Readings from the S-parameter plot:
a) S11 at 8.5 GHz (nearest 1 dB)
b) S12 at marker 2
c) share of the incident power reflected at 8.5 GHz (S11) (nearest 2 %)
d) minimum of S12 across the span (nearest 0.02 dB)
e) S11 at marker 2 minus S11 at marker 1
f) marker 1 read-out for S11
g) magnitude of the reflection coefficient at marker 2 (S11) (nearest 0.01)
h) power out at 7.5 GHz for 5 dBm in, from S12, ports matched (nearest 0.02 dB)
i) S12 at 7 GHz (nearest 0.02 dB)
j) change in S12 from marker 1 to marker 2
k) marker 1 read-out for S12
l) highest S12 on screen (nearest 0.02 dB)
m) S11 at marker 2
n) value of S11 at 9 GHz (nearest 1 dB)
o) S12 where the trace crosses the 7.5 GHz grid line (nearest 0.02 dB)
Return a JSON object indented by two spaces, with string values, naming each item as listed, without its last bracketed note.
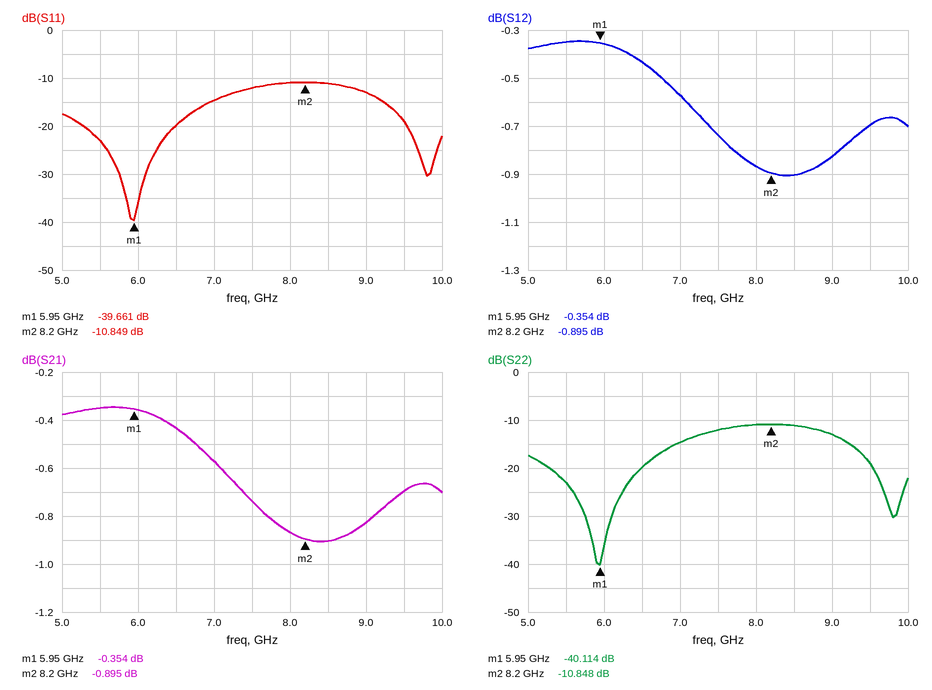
{
  "S11 at 8.5 GHz": "-11 dB",
  "S12 at marker 2": "-0.895 dB",
  "share of the incident power reflected at 8.5 GHz (S11)": "8 %",
  "minimum of S12 across the span": "-0.90 dB",
  "S11 at marker 2 minus S11 at marker 1": "28.812 dB",
  "marker 1 read-out for S11": "-39.661 dB",
  "magnitude of the reflection coefficient at marker 2 (S11)": "0.29",
  "power out at 7.5 GHz for 5 dBm in, from S12, ports matched": "4.26 dBm",
  "S12 at 7 GHz": "-0.58 dB",
  "change in S12 from marker 1 to marker 2": "-0.541 dB",
  "marker 1 read-out for S12": "-0.354 dB",
  "highest S12 on screen": "-0.34 dB",
  "S11 at marker 2": "-10.849 dB",
  "value of S11 at 9 GHz": "-13 dB",
  "S12 where the trace crosses the 7.5 GHz grid line": "-0.74 dB"
}
